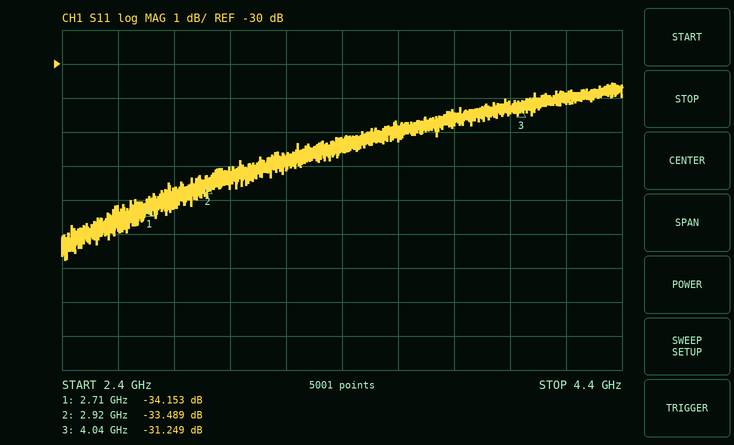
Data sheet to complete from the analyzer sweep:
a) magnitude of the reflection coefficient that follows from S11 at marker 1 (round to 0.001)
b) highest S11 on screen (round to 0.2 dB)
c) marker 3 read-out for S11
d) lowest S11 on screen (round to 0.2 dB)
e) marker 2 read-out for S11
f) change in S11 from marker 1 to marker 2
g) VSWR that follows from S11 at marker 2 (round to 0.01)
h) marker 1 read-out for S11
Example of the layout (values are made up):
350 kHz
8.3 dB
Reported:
0.020
-30.6 dB
-31.249 dB
-35.8 dB
-33.489 dB
0.664 dB
1.04
-34.153 dB
